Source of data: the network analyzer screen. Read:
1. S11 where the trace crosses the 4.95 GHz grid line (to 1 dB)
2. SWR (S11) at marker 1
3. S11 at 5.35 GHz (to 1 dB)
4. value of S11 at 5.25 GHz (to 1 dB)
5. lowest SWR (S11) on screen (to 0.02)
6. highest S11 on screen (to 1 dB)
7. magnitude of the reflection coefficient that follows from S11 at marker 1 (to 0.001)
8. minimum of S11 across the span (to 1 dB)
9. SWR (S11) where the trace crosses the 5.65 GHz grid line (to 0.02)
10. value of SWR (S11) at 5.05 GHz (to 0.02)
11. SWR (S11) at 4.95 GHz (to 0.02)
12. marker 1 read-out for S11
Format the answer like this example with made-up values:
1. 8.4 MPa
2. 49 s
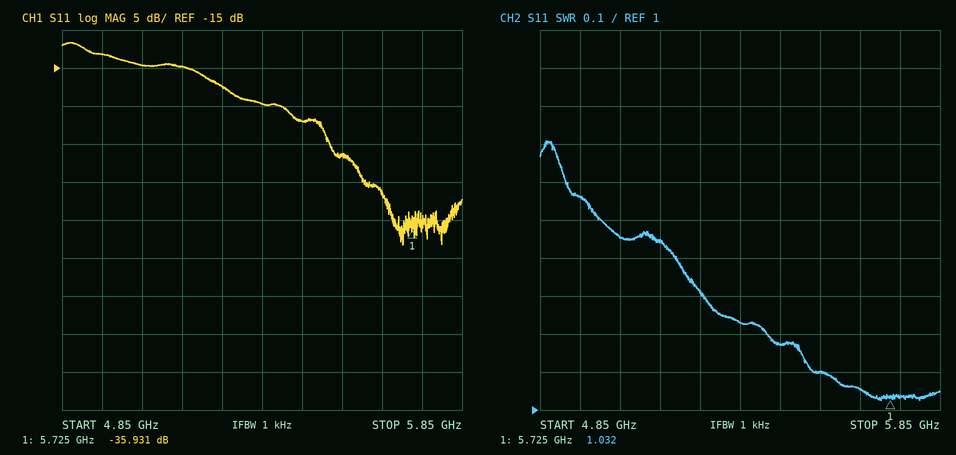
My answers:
1. -13 dB
2. 1.032
3. -20 dB
4. -17 dB
5. 1.02
6. -12 dB
7. 0.016
8. -38 dB
9. 1.06
10. 1.46
11. 1.56
12. -35.931 dB
